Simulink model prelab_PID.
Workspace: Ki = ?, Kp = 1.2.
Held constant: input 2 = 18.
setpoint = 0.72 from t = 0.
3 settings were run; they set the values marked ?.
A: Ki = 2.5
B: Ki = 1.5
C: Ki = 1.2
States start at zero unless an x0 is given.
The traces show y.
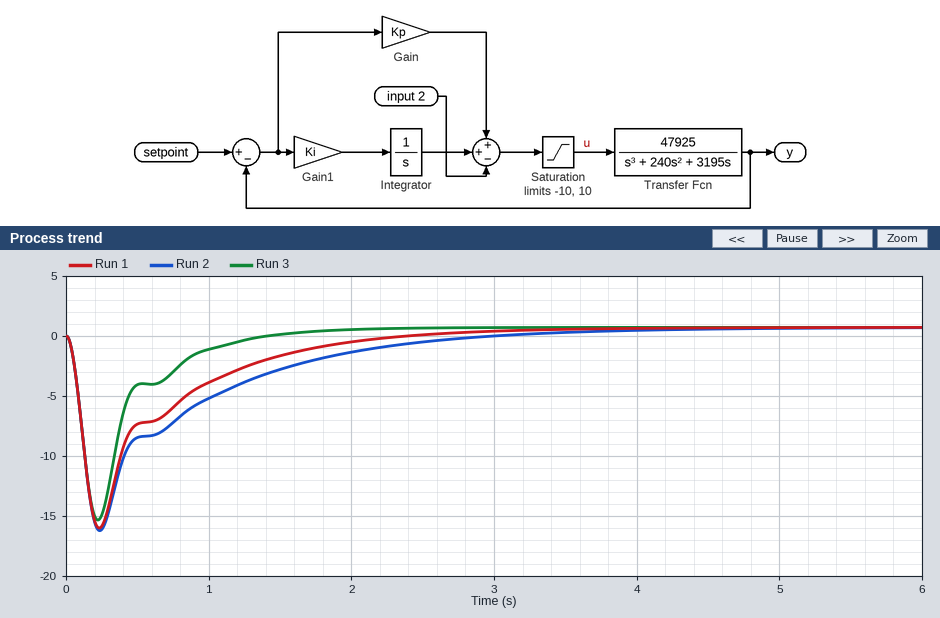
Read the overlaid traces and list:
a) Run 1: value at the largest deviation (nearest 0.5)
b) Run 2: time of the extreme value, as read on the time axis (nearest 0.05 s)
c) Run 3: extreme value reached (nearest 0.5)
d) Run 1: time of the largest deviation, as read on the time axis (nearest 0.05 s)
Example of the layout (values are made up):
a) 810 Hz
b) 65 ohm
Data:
a) -16.0
b) 0.25 s
c) -15.5
d) 0.25 s
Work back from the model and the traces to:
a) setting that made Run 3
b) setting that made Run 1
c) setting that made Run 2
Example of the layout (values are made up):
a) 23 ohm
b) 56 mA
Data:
a) A
b) B
c) C
